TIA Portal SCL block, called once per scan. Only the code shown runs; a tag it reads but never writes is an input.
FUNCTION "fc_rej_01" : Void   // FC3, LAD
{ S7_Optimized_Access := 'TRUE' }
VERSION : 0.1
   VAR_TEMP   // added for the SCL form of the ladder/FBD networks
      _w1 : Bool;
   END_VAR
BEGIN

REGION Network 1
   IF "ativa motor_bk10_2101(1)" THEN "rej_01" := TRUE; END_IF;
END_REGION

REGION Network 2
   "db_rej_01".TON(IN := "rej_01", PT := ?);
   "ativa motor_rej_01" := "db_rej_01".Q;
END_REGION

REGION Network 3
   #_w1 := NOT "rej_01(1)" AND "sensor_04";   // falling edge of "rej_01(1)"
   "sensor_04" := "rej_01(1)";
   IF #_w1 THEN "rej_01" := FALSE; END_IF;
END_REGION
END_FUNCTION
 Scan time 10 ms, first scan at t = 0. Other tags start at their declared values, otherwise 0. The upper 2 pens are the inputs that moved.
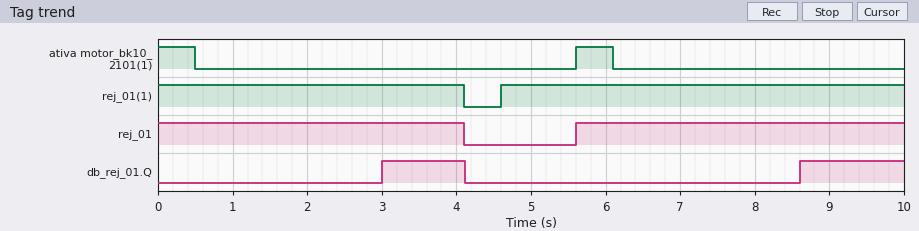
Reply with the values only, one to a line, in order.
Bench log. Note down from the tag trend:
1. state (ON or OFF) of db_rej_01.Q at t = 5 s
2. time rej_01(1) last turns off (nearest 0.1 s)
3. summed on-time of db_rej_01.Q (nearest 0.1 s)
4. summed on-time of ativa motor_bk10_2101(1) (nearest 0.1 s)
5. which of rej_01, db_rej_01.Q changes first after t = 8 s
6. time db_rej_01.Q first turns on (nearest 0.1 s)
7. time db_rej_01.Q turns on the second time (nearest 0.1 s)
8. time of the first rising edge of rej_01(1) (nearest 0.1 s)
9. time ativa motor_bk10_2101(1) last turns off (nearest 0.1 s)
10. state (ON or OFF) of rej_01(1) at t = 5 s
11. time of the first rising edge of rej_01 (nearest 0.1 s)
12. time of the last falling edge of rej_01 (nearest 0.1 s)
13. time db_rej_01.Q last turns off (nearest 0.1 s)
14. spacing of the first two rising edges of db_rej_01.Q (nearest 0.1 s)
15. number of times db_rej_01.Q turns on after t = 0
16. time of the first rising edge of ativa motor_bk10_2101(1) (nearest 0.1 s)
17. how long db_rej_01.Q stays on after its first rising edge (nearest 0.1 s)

OFF
4.1 s
2.5 s
1.0 s
db_rej_01.Q
3.0 s
8.6 s
4.6 s
6.1 s
ON
5.6 s
4.1 s
4.1 s
5.6 s
2
5.6 s
1.1 s
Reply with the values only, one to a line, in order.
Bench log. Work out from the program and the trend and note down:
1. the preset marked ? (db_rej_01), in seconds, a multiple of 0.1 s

3.0 s
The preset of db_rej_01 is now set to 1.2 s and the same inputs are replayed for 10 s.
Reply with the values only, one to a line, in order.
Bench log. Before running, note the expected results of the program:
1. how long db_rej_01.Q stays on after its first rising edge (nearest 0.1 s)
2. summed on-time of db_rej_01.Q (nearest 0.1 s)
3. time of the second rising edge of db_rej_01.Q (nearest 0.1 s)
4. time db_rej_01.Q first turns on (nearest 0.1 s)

2.9 s
6.1 s
6.8 s
1.2 s
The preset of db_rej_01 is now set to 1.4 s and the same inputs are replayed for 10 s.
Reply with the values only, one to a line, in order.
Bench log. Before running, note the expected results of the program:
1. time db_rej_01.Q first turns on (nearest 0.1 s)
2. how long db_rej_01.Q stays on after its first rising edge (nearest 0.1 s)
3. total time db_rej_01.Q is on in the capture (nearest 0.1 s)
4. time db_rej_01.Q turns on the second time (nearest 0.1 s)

1.4 s
2.7 s
5.7 s
7.0 s
